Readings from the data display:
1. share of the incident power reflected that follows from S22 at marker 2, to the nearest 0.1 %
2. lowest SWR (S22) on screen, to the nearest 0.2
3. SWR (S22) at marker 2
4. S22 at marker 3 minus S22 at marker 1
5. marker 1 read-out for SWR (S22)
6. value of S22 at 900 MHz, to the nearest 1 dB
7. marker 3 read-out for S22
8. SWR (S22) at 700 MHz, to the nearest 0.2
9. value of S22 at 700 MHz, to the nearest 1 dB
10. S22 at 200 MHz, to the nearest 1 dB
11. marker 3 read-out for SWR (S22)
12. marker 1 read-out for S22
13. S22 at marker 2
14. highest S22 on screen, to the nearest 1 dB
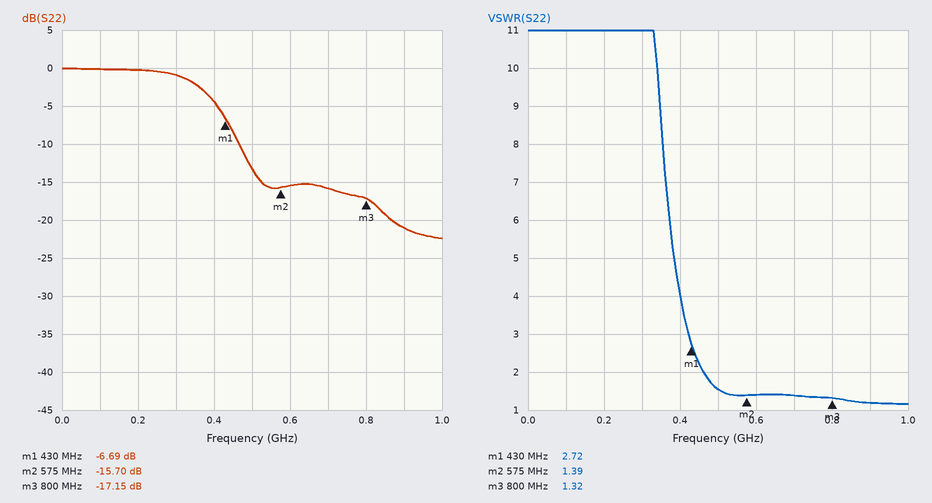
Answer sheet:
2.7 %
1.2
1.39
-10.46 dB
2.72
-21 dB
-17.15 dB
1.4
-16 dB
0 dB
1.32
-6.69 dB
-15.70 dB
0 dB
